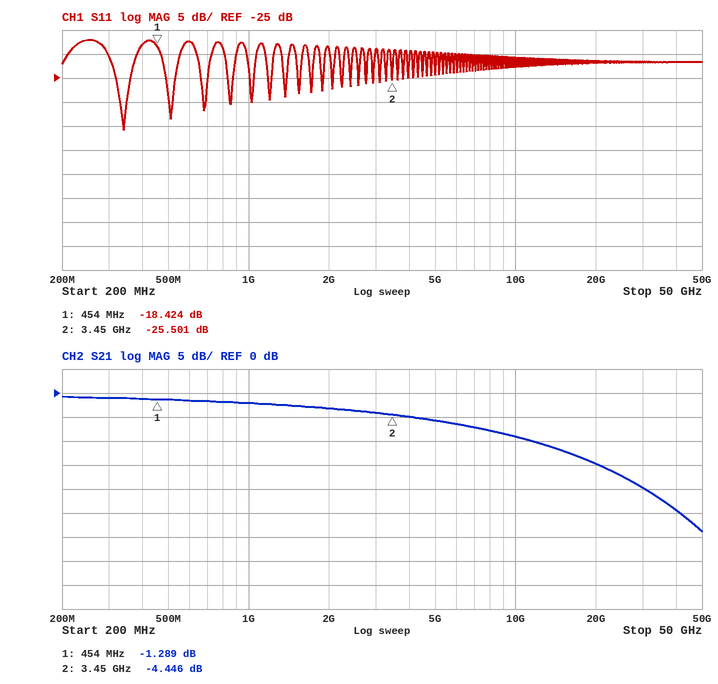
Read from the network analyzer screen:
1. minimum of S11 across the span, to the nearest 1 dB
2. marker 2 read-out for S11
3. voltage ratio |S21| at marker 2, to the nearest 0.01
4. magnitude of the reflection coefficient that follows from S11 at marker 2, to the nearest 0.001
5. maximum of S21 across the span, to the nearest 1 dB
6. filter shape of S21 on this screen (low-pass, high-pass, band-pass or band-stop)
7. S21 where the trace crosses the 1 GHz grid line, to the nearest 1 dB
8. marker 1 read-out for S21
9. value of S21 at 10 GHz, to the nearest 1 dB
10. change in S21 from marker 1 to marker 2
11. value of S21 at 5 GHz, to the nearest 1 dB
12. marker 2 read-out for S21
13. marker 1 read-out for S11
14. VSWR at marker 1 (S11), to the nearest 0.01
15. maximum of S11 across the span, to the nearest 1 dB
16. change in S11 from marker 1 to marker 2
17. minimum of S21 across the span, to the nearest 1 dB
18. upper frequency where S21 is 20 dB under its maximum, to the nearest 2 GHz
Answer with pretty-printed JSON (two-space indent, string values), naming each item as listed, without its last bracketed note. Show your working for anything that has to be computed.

{
  "minimum of S11 across the span, to the nearest 1 dB": "-36 dB",
  "marker 2 read-out for S11": "-25.501 dB",
  "voltage ratio |S21| at marker 2, to the nearest 0.01": "10^(-4.446/20) ≈ 0.60",
  "magnitude of the reflection coefficient that follows from S11 at marker 2, to the nearest 0.001": "10^(-25.501/20) ≈ 0.053",
  "maximum of S21 across the span, to the nearest 1 dB": "-1 dB",
  "filter shape of S21 on this screen": "low-pass",
  "S21 where the trace crosses the 1 GHz grid line, to the nearest 1 dB": "-2 dB",
  "marker 1 read-out for S21": "-1.289 dB",
  "value of S21 at 10 GHz, to the nearest 1 dB": "-9 dB",
  "change in S21 from marker 1 to marker 2": "-4.446 − (-1.289) = -3.157 dB",
  "value of S21 at 5 GHz, to the nearest 1 dB": "-6 dB",
  "marker 2 read-out for S21": "-4.446 dB",
  "marker 1 read-out for S11": "-18.424 dB",
  "VSWR at marker 1 (S11), to the nearest 0.01": "(1 + 0.1199)/(1 − 0.1199) ≈ 1.27",
  "maximum of S11 across the span, to the nearest 1 dB": "-17 dB",
  "change in S11 from marker 1 to marker 2": "-25.501 − (-18.424) = -7.077 dB",
  "minimum of S21 across the span, to the nearest 1 dB": "-29 dB",
  "upper frequency where S21 is 20 dB under its maximum, to the nearest 2 GHz": "32 GHz"
}
